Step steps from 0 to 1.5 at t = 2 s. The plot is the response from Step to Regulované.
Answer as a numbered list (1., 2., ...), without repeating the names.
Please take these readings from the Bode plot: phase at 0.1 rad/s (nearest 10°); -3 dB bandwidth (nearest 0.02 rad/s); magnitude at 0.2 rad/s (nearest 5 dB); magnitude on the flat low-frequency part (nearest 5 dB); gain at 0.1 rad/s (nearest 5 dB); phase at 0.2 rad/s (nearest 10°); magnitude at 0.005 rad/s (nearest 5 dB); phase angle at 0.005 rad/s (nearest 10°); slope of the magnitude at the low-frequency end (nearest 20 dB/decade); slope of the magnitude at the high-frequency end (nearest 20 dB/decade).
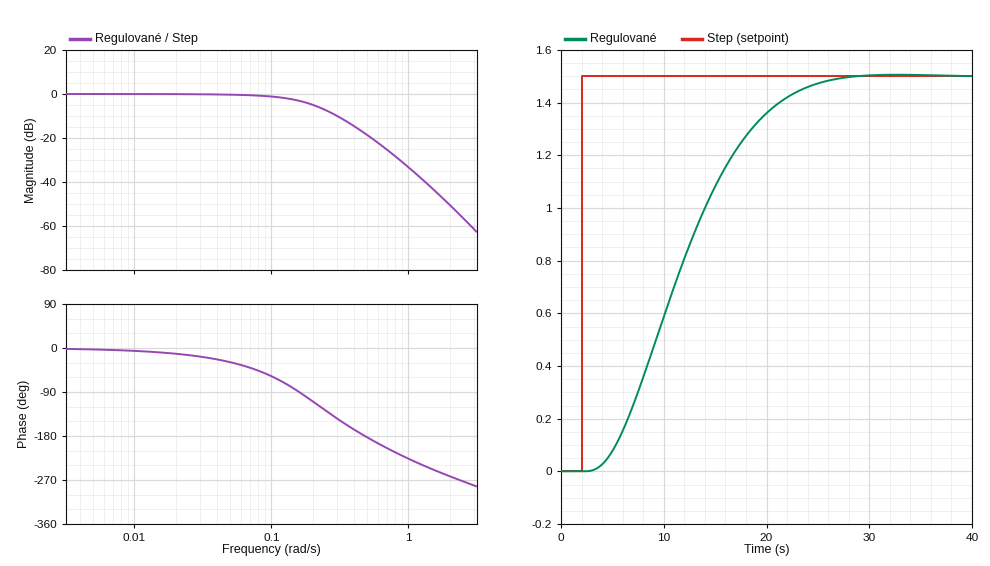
1. -60°
2. 0.16 rad/s
3. -5 dB
4. 0 dB
5. 0 dB
6. -110°
7. 0 dB
8. 0°
9. 0 dB/decade
10. -60 dB/decade
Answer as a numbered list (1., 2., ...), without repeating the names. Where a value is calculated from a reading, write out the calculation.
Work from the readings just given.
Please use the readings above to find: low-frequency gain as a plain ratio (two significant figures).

1. 10^(0 / 20) = 1.0
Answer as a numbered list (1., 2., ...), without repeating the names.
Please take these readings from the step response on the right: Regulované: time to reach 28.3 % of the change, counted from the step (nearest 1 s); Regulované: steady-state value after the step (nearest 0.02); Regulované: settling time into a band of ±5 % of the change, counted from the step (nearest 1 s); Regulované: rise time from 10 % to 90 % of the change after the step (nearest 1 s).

1. 7 s
2. 1.50
3. 20 s
4. 14 s
